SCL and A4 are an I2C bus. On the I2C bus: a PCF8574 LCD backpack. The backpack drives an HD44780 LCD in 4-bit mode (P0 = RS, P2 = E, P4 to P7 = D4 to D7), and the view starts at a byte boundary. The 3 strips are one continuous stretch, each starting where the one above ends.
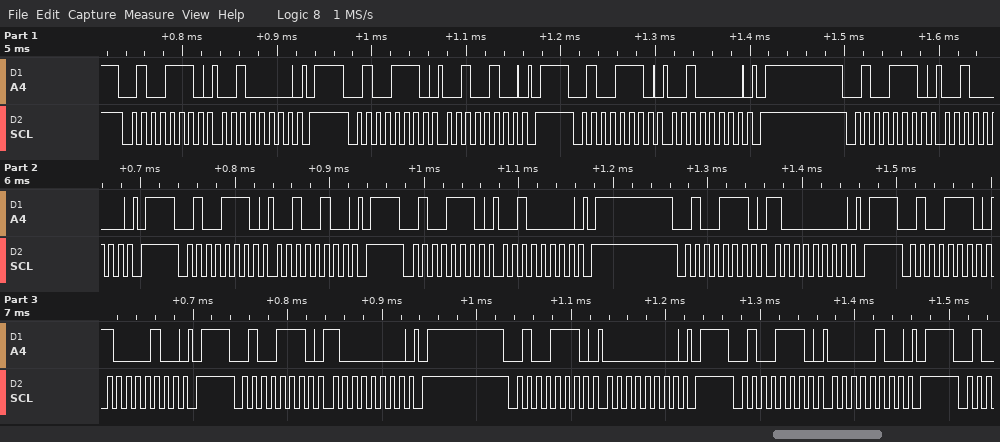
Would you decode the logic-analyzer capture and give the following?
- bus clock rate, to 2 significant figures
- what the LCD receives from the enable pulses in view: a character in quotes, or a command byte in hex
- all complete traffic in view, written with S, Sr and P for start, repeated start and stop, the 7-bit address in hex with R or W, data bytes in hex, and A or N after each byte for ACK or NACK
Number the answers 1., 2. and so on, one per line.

1. 100 kHz
2. 0x28
3. S 27W A 20 A P S 27W A 24 A P S 27W A 20 A P S 27W A 20 A P S 27W A 24 A P S 27W A 20 A P S 27W A 80 A P S 27W A 84 A P S 27W A 80 A P S 27W A 00 A P S 27W A 04 A P
